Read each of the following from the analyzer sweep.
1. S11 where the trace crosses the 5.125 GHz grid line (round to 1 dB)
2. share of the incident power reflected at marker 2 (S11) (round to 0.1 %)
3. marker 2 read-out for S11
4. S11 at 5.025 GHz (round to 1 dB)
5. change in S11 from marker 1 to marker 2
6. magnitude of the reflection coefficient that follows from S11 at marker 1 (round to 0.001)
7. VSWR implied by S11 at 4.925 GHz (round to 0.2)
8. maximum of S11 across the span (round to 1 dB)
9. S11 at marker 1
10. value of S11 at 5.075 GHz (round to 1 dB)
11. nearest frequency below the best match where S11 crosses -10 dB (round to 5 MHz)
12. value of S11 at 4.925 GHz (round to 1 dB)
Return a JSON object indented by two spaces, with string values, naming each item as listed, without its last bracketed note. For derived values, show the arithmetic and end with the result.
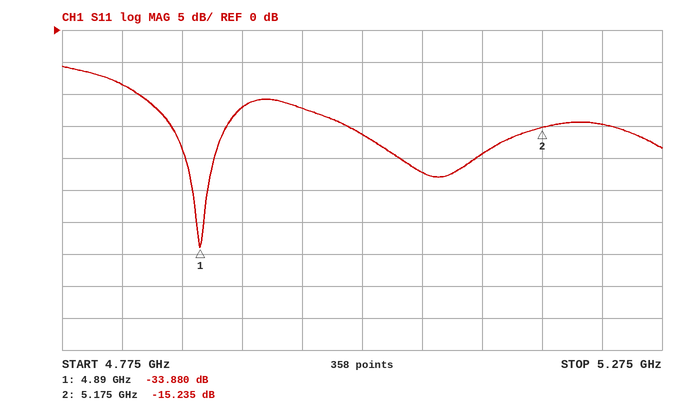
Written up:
{
  "S11 where the trace crosses the 5.125 GHz grid line": "-19 dB",
  "share of the incident power reflected at marker 2 (S11)": "10^(-15.235/10) ≈ 3.0 %",
  "marker 2 read-out for S11": "-15.235 dB",
  "S11 at 5.025 GHz": "-16 dB",
  "change in S11 from marker 1 to marker 2": "-15.235 − (-33.88) = 18.645 dB",
  "magnitude of the reflection coefficient that follows from S11 at marker 1": "10^(-33.88/20) ≈ 0.020",
  "VSWR implied by S11 at 4.925 GHz": "|Γ| = 10^(-12/20) = 0.2512; VSWR = (1 + 0.2512)/(1 − 0.2512) ≈ 1.67, so 1.6 to the nearest 0.2",
  "maximum of S11 across the span": "-6 dB",
  "S11 at marker 1": "-33.880 dB",
  "value of S11 at 5.075 GHz": "-22 dB",
  "nearest frequency below the best match where S11 crosses -10 dB": "4.840 GHz",
  "value of S11 at 4.925 GHz": "-12 dB"
}
